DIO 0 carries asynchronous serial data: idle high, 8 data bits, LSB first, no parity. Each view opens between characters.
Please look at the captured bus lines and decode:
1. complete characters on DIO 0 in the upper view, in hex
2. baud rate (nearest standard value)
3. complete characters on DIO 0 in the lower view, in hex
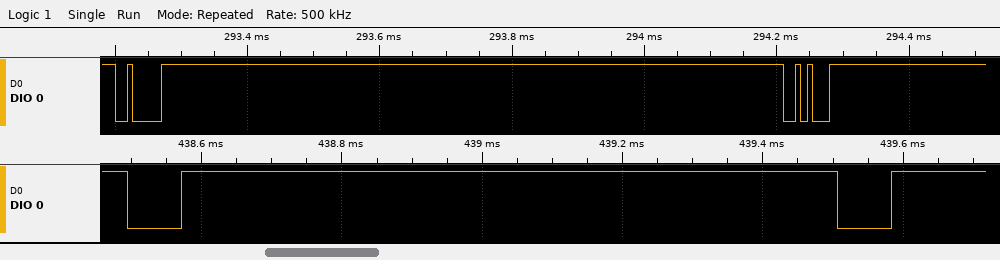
82, 8A
115200 baud
00, 00
